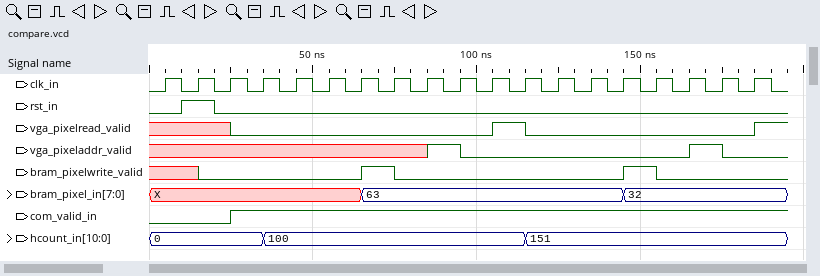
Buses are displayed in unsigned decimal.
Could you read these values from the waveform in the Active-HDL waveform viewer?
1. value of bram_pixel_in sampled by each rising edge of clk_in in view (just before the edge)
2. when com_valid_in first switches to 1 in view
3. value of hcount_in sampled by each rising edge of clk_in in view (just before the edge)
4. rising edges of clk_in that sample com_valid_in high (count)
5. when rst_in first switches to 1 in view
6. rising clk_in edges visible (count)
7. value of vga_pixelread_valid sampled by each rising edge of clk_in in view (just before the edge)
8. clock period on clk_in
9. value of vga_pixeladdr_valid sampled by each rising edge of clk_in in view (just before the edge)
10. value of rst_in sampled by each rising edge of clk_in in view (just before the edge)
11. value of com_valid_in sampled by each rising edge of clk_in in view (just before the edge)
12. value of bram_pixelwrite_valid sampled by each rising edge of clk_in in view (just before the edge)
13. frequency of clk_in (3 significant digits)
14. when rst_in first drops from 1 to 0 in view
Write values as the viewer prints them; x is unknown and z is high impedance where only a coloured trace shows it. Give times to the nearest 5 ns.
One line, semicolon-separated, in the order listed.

X, X, X, X, X, X, X, 63, 63, 63, 63, 63, 63, 63, 63, 32, 32, 32, 32; 25 ns; 0, 0, 0, 0, 100, 100, 100, 100, 100, 100, 100, 100, 151, 151, 151, 151, 151, 151, 151; 16; 10 ns; 19; x x x 0 0 0 0 0 0 0 0 1 0 0 0 0 0 0 0; 10 ns; x x x x x x x x x 1 0 0 0 0 0 0 0 1 0; 0 1 0 0 0 0 0 0 0 0 0 0 0 0 0 0 0 0 0; 0 0 0 1 1 1 1 1 1 1 1 1 1 1 1 1 1 1 1; x x 0 0 0 0 0 1 0 0 0 0 0 0 0 1 0 0 0; 100 MHz; 20 ns
